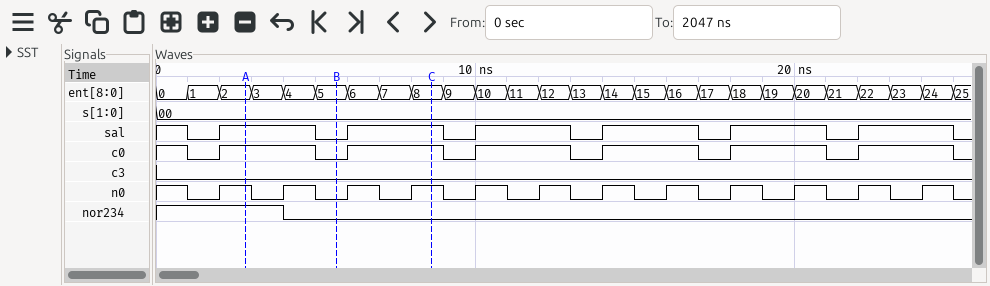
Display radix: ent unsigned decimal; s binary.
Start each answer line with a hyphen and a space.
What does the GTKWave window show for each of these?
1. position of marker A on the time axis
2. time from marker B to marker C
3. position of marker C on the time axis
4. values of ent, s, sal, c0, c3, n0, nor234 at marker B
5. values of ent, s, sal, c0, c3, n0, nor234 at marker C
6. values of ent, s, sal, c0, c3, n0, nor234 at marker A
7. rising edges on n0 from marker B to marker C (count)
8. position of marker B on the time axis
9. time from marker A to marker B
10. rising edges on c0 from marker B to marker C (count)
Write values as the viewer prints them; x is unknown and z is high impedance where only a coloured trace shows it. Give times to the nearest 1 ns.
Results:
- 3 ns
- 3 ns
- 9 ns
- ent=5, s=00, sal=0, c0=0, c3=0, n0=0, nor234=0
- ent=8, s=00, sal=1, c0=1, c3=0, n0=1, nor234=0
- ent=2, s=00, sal=1, c0=1, c3=0, n0=1, nor234=1
- 2
- 6 ns
- 3 ns
- 1
